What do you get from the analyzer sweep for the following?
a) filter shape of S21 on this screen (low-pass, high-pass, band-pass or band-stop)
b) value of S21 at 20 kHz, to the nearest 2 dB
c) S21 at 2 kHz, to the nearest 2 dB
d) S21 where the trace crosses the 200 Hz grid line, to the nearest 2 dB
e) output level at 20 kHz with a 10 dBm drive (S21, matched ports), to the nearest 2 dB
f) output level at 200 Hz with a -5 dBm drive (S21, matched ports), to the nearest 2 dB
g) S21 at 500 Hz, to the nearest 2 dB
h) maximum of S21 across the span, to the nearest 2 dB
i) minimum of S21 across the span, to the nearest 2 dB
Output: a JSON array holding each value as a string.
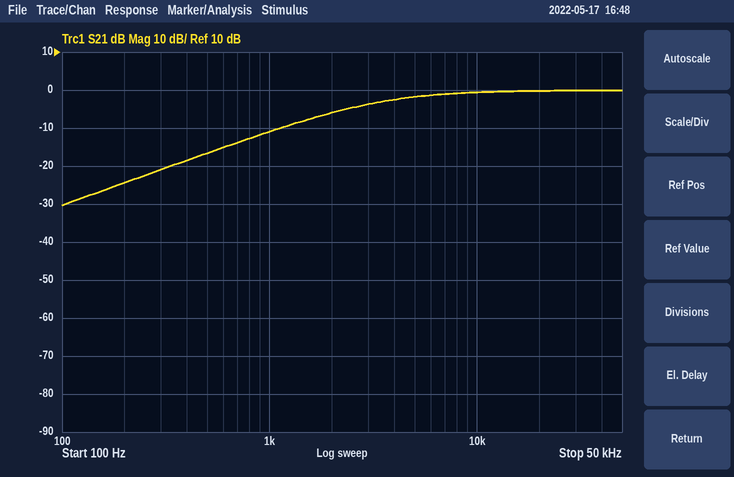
["high-pass", "0 dB", "-6 dB", "-24 dB", "10 dBm", "-30 dBm", "-16 dB", "0 dB", "-30 dB"]
